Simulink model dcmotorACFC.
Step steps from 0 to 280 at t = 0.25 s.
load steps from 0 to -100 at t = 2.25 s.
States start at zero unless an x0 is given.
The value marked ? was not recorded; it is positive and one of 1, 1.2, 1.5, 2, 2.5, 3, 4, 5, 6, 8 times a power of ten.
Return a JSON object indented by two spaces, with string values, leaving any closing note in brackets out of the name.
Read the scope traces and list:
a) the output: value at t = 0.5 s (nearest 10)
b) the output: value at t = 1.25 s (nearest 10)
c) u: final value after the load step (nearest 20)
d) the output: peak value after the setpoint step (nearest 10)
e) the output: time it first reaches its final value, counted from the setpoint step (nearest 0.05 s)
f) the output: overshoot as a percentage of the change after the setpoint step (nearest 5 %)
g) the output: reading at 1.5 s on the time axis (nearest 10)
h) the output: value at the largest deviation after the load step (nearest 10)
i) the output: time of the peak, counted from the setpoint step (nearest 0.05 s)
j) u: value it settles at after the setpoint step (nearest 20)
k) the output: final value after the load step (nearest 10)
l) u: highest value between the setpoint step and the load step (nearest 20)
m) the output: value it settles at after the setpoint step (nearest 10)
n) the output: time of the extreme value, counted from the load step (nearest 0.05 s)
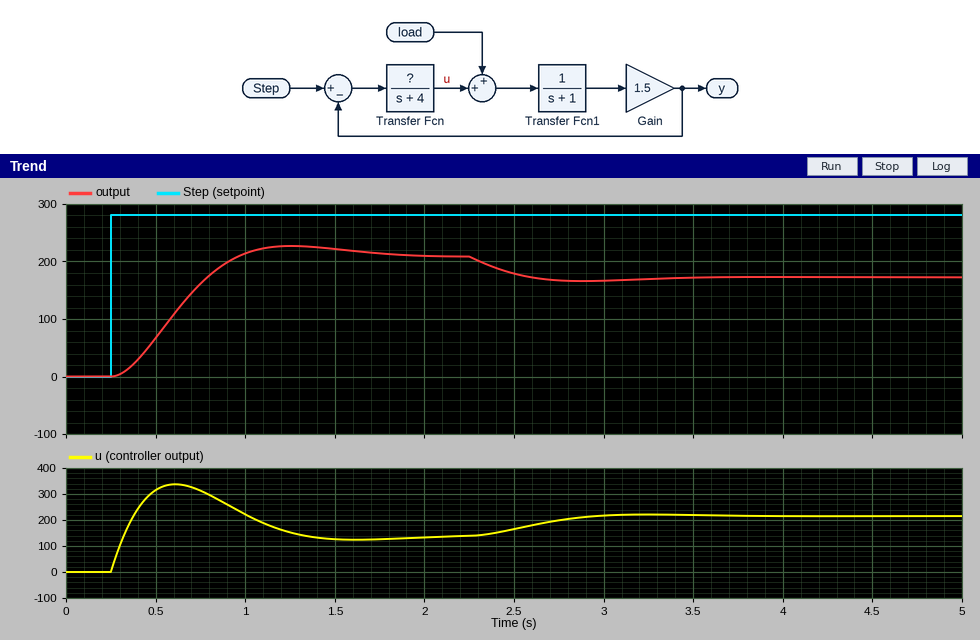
{
  "the output: value at t = 0.5 s": "70",
  "the output: value at t = 1.25 s": "230",
  "u: final value after the load step": "220",
  "the output: peak value after the setpoint step": "230",
  "the output: time it first reaches its final value, counted from the setpoint step": "0.70 s",
  "the output: overshoot as a percentage of the change after the setpoint step": "10 %",
  "the output: reading at 1.5 s on the time axis": "220",
  "the output: value at the largest deviation after the load step": "170",
  "the output: time of the peak, counted from the setpoint step": "1.00 s",
  "u: value it settles at after the setpoint step": "140",
  "the output: final value after the load step": "170",
  "u: highest value between the setpoint step and the load step": "340",
  "the output: value it settles at after the setpoint step": "210",
  "the output: time of the extreme value, counted from the load step": "0.65 s"
}
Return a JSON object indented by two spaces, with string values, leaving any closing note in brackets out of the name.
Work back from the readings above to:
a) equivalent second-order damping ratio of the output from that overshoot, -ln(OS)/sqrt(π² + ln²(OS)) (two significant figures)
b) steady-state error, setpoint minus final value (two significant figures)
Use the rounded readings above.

{
  "equivalent second-order damping ratio of the output from that overshoot, -ln(OS)/sqrt(π² + ln²(OS))": "0.59",
  "steady-state error, setpoint minus final value": "70"
}
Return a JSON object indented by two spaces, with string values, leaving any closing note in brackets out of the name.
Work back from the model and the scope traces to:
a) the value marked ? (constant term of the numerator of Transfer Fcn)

{
  "the value marked ?": "8"
}
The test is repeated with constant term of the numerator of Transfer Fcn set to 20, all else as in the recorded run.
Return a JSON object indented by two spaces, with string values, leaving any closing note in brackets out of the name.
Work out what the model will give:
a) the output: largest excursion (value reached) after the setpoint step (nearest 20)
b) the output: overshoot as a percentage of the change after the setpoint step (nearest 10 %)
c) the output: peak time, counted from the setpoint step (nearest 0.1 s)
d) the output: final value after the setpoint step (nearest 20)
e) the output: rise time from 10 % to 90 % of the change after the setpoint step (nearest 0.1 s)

{
  "the output: largest excursion (value reached) after the setpoint step": "300",
  "the output: overshoot as a percentage of the change after the setpoint step": "20 %",
  "the output: peak time, counted from the setpoint step": "0.6 s",
  "the output: final value after the setpoint step": "240",
  "the output: rise time from 10 % to 90 % of the change after the setpoint step": "0.3 s"
}
